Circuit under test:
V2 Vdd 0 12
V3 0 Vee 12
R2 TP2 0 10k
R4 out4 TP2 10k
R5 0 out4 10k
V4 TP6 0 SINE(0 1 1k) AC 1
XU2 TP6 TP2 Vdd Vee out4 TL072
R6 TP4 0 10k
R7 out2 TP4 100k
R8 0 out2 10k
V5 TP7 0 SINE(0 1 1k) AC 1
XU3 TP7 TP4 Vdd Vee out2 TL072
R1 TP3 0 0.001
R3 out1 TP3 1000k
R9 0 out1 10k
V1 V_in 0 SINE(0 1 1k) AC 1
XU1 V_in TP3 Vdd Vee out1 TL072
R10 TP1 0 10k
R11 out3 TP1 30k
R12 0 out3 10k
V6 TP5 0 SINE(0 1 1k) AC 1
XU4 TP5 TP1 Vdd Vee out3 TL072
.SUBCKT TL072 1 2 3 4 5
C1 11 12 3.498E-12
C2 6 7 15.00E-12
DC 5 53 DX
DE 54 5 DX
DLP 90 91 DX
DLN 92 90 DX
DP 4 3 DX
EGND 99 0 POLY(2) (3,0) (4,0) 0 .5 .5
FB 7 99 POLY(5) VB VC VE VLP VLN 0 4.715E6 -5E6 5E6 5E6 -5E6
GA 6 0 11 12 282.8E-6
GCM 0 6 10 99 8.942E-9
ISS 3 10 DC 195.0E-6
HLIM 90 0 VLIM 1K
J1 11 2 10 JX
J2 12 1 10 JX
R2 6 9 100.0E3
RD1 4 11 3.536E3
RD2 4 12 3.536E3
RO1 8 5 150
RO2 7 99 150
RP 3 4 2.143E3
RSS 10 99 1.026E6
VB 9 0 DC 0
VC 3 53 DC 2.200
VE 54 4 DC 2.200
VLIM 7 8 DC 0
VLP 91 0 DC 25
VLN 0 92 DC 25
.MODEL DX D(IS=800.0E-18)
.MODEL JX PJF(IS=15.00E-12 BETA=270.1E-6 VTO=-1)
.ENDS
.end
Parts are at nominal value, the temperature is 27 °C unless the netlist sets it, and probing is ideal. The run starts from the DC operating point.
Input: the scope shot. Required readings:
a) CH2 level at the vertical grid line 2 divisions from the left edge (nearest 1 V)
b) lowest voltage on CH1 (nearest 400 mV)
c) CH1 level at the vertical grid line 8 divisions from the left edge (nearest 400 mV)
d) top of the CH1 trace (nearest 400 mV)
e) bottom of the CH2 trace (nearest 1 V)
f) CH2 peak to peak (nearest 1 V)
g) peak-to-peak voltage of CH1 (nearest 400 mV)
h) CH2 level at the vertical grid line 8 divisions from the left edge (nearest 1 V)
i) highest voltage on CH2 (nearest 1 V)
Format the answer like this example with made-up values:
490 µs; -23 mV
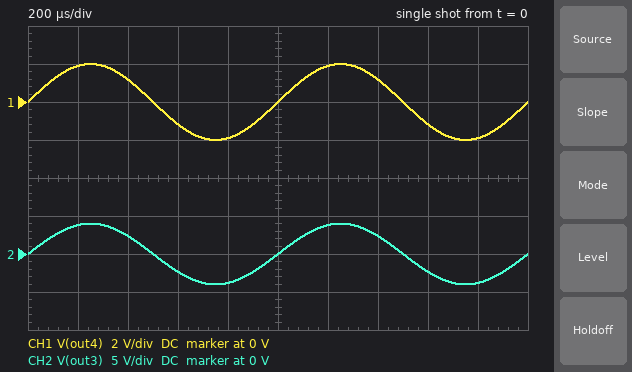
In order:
2 V; -2.0 V; -1.2 V; 2.0 V; -4 V; 8 V; 4.0 V; -2 V; 4 V
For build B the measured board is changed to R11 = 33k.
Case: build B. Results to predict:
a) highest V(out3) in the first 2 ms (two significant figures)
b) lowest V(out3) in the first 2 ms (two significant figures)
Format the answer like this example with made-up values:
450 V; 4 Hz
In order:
4.3 V; -4.3 V
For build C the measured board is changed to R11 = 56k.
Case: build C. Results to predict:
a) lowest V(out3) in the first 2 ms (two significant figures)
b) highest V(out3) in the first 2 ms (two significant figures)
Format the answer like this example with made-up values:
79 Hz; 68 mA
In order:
-6.6 V; 6.6 V
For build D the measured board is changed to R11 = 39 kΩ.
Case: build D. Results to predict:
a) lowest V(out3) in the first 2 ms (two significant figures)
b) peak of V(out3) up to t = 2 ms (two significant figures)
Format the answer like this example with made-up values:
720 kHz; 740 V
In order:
-4.9 V; 4.9 V
